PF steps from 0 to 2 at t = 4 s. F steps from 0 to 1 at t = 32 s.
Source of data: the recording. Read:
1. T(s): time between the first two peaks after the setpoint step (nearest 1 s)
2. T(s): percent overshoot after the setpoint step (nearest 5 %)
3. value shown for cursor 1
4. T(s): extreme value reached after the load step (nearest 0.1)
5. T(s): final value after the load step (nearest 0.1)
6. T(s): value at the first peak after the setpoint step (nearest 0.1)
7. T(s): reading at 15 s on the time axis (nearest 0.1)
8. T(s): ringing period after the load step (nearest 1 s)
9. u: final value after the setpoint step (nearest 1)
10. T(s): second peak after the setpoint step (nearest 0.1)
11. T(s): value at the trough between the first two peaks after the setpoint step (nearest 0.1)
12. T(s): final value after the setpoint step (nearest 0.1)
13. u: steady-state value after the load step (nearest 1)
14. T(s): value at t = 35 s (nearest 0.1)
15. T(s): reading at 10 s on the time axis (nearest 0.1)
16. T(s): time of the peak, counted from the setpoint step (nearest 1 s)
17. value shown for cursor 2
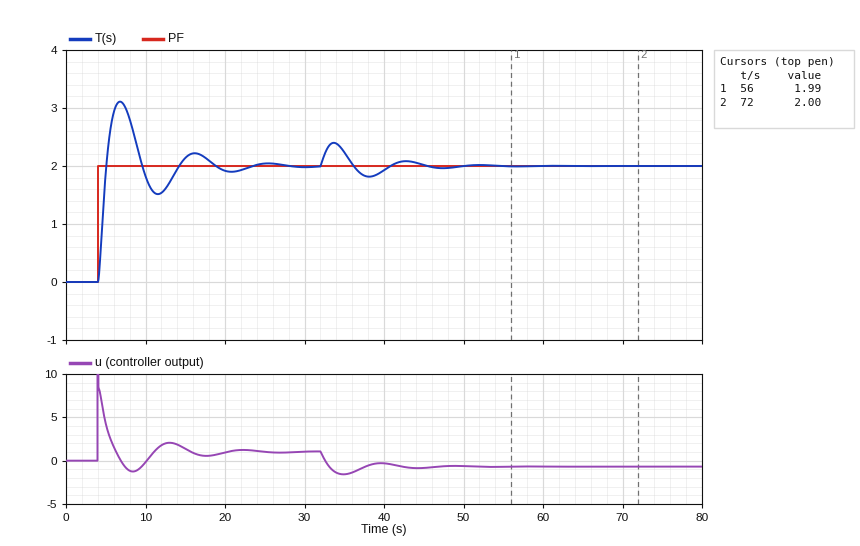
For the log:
9 s
55 %
1.99
2.4
2.0
3.1
2.1
9 s
1
2.2
1.5
2.0
-1
2.2
1.8
3 s
2.00
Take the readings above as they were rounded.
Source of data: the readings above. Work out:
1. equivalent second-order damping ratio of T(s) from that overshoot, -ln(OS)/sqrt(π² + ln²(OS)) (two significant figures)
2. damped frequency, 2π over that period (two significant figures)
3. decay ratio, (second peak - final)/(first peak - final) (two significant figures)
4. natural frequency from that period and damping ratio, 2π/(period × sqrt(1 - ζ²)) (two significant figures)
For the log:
0.19
0.70 rad/s
0.18
0.71 rad/s
